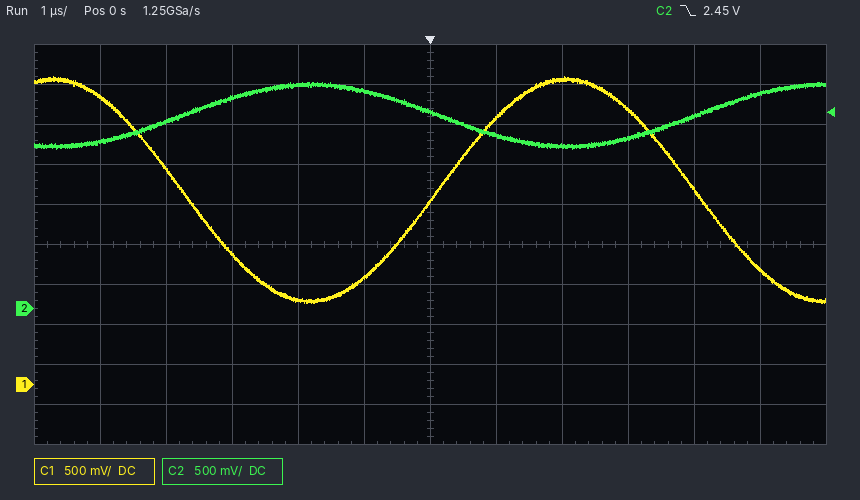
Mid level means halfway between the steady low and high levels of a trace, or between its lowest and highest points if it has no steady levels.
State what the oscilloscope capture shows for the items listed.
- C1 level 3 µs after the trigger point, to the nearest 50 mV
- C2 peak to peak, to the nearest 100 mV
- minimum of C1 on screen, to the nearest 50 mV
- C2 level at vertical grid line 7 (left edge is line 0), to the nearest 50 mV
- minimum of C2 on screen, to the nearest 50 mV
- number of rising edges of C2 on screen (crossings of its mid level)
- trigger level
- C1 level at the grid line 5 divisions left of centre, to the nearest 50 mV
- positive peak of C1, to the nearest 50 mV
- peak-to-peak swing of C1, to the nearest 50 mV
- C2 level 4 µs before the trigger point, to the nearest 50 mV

3.45 V
800 mV
1.00 V
2.15 V
2.00 V
2
2.45 V
3.60 V
3.85 V
2.85 V
2.35 V
